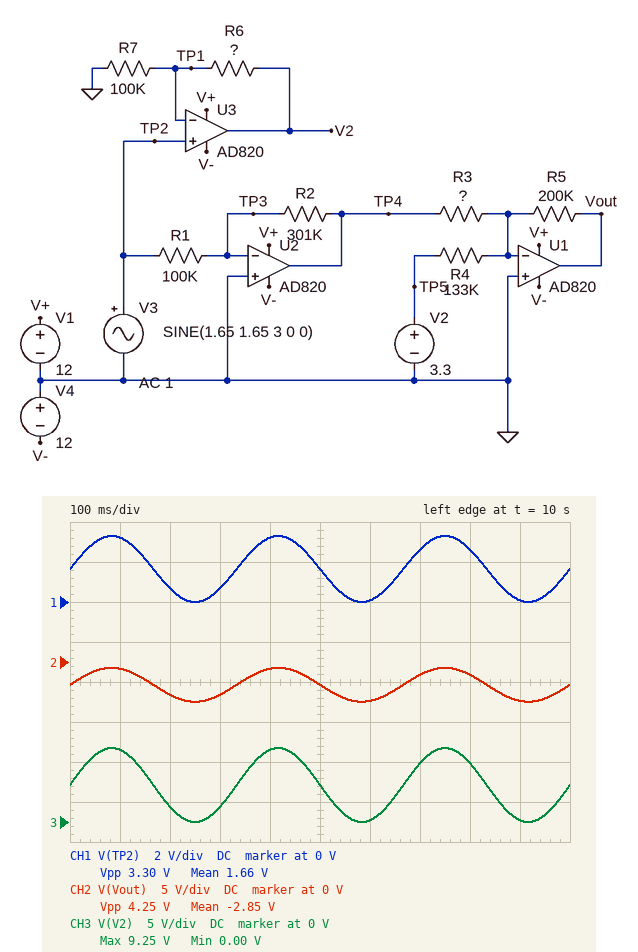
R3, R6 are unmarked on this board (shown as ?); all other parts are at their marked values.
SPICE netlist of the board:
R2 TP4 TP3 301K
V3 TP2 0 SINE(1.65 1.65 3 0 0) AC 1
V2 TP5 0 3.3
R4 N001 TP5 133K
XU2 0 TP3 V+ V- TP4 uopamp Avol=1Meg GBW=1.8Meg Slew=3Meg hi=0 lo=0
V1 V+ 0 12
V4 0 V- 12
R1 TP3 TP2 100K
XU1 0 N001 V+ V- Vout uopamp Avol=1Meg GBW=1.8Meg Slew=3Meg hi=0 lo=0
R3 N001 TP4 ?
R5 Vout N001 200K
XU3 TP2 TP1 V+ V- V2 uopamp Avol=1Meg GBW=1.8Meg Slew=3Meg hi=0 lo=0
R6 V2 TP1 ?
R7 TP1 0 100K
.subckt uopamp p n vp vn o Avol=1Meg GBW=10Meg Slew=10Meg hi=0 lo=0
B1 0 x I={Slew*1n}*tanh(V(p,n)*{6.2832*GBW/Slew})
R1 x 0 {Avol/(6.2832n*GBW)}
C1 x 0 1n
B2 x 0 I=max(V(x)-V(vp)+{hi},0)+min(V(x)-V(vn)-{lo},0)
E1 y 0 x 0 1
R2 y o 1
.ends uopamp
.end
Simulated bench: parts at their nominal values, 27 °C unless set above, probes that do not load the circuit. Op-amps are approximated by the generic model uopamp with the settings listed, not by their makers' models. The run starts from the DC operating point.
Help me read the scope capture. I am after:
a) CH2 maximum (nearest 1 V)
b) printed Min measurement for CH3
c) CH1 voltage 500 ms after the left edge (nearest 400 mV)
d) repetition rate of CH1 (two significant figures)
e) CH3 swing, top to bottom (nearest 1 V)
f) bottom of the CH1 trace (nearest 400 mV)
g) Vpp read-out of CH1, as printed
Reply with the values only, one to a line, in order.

-1 V
0.00 V
1.6 V
3.0 Hz
9 V
0 V
3.30 V
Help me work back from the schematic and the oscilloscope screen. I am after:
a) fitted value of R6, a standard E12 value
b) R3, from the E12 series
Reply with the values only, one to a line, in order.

180 kΩ
470 kΩ
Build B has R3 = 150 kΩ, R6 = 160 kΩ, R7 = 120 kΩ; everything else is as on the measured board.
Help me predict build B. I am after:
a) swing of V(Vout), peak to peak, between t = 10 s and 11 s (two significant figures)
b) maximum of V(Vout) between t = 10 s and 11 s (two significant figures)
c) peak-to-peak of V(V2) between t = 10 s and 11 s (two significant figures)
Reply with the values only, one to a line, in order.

13 V
8.3 V
7.7 V
